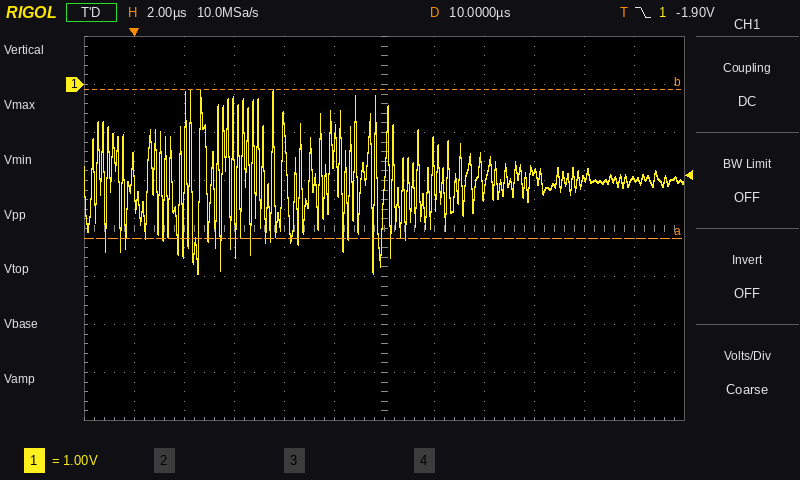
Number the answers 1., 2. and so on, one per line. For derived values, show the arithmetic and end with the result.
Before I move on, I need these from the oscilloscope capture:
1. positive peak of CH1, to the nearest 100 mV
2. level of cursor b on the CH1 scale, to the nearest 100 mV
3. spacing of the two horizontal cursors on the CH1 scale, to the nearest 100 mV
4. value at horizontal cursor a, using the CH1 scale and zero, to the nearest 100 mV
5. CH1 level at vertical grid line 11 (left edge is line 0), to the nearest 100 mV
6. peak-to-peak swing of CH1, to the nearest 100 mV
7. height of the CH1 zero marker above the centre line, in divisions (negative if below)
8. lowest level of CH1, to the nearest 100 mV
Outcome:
1. -100 mV
2. -100 mV
3. 3.1 V
4. -3.2 V
5. -2.0 V
6. -100 mV − (-3.9 V) = 3.8 V
7. +3.0 div
8. -3.9 V
